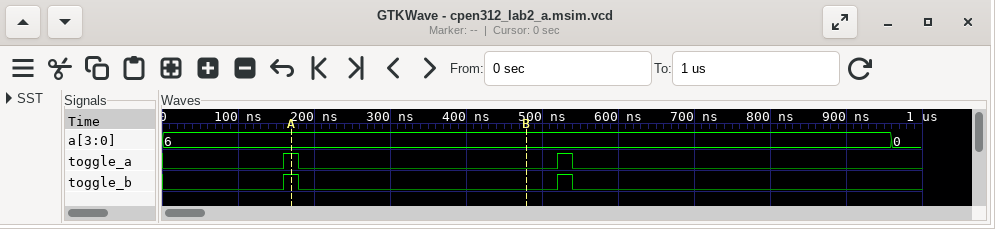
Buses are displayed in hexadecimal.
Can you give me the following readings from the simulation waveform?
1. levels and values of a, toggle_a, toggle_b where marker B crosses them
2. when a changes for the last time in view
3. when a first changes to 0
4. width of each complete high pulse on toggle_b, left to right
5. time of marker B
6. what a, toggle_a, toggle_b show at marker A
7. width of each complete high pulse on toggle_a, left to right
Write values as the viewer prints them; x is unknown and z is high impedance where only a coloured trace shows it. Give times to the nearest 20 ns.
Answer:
a=6, toggle_a=0, toggle_b=0
960 ns
960 ns
20 ns, 20 ns
480 ns
a=6, toggle_a=1, toggle_b=1
20 ns, 20 ns
